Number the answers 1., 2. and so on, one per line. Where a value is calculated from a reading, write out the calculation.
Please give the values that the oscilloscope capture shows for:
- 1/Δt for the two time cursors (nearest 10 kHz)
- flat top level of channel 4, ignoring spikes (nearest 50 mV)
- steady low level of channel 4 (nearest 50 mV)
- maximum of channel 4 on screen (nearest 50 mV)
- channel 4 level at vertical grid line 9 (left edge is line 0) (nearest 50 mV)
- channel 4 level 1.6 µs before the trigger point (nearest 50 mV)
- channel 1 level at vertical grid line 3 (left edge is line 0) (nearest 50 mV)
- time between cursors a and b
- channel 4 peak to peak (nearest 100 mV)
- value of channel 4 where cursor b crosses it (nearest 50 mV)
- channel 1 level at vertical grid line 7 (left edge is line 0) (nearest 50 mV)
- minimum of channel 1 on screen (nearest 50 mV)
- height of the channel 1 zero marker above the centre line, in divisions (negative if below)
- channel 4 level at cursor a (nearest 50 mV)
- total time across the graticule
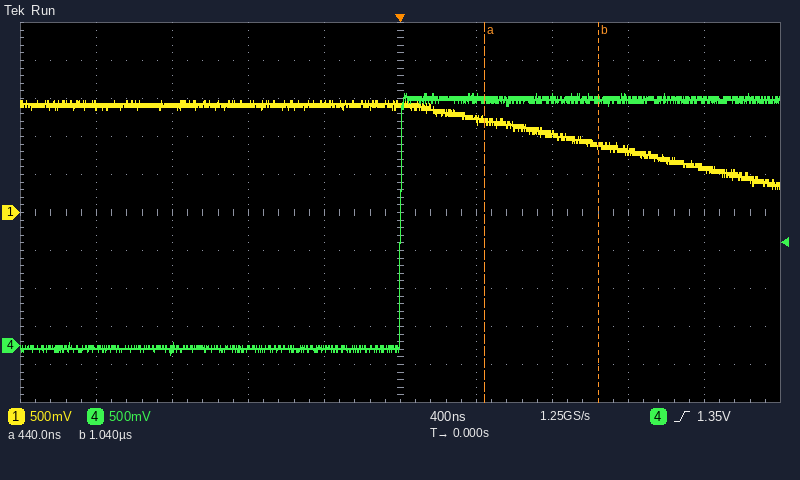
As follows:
1. 1 / 600 ns ≈ 1.67 MHz
2. 3.25 V
3. -50 mV
4. 3.30 V
5. 3.25 V
6. -50 mV
7. 1.45 V
8. 1.04 µs − (440 ns) = 600 ns
9. 3.40 V
10. 3.25 V
11. 1.05 V
12. 300 mV
13. 0.0 div
14. 3.25 V
15. 4 µs
